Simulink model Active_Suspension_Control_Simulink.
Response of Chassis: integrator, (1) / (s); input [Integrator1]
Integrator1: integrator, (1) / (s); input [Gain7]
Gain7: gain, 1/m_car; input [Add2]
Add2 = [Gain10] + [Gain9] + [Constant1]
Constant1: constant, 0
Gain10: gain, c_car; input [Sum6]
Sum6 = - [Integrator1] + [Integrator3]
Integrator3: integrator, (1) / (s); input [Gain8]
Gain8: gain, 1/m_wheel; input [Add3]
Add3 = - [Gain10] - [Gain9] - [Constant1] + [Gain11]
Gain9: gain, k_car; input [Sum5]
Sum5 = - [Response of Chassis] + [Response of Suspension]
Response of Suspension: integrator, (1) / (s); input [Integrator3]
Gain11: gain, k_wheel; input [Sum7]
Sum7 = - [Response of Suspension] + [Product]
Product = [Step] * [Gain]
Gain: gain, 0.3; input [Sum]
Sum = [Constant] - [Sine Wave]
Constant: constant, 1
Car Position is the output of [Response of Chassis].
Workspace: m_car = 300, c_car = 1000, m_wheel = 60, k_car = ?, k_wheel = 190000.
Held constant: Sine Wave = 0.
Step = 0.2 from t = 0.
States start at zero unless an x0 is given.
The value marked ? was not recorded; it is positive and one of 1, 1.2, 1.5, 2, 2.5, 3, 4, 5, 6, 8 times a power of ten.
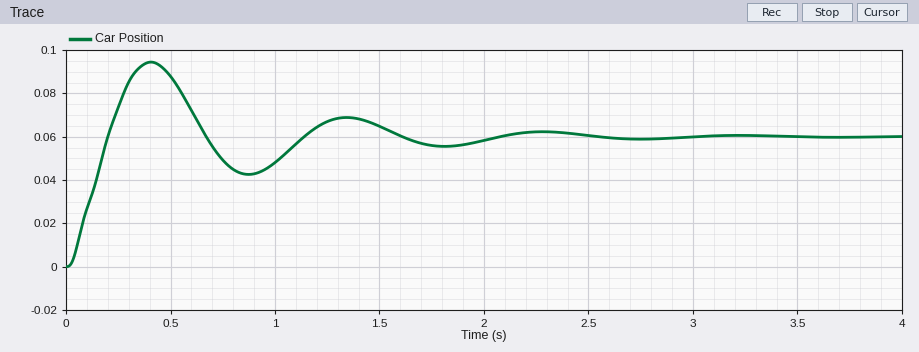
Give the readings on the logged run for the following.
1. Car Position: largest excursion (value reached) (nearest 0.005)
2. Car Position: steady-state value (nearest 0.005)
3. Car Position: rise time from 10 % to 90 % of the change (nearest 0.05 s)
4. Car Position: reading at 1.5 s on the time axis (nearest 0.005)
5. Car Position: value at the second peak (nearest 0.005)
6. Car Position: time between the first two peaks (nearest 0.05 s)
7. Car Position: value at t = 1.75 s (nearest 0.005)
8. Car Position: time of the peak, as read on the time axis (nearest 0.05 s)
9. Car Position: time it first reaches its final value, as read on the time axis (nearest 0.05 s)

0.095
0.060
0.15 s
0.065
0.070
0.95 s
0.055
0.40 s
0.20 s
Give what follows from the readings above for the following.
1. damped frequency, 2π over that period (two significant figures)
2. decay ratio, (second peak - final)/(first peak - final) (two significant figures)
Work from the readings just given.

6.6 rad/s
0.29
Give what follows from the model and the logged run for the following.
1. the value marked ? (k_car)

15000
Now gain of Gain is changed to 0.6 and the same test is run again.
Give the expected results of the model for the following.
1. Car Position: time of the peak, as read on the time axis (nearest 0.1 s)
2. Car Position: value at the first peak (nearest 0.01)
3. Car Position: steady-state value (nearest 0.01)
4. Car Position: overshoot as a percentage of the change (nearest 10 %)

0.4 s
0.19
0.12
60 %
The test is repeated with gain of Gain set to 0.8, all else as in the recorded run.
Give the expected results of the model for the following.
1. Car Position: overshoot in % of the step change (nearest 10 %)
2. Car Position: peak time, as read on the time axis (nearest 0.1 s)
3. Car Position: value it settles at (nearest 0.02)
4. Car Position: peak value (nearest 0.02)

60 %
0.4 s
0.16
0.26
